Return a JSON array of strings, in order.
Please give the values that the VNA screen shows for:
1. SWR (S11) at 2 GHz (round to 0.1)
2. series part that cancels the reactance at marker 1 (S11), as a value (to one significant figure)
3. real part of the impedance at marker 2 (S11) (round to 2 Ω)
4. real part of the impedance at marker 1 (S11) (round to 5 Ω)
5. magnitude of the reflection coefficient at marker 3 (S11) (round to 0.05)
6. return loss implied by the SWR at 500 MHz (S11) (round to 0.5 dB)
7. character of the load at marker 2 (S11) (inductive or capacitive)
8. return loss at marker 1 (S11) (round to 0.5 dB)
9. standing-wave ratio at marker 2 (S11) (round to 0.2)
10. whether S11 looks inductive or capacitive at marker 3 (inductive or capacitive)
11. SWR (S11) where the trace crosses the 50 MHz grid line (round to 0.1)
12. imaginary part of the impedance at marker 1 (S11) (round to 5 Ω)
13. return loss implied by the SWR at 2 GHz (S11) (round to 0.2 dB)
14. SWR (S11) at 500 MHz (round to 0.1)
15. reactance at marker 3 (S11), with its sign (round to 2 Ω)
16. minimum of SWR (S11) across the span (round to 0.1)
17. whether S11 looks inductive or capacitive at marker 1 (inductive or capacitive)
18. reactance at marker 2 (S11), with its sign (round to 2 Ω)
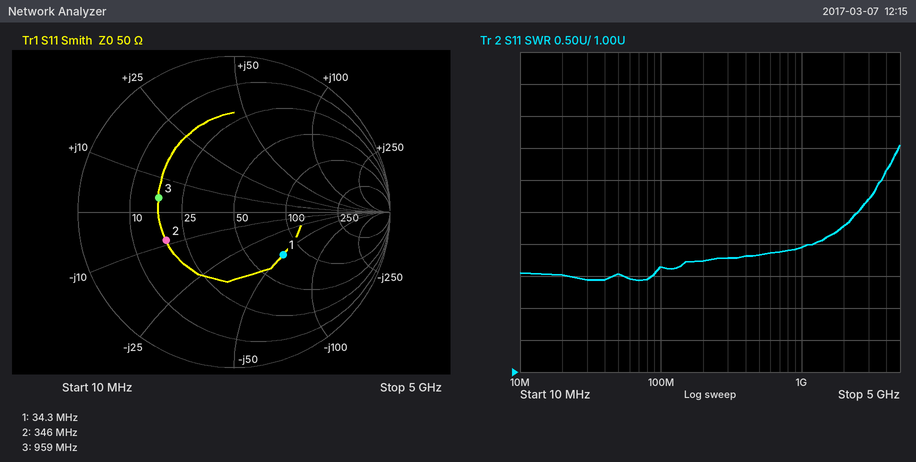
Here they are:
["3.3", "200 nH", "18 Ω", "75 Ω", "0.50", "6.5 dB", "capacitive", "7.5 dB", "2.8", "inductive", "2.5", "-50 Ω", "5.4 dB", "2.8", "+4 Ω", "2.4", "capacitive", "-8 Ω"]
